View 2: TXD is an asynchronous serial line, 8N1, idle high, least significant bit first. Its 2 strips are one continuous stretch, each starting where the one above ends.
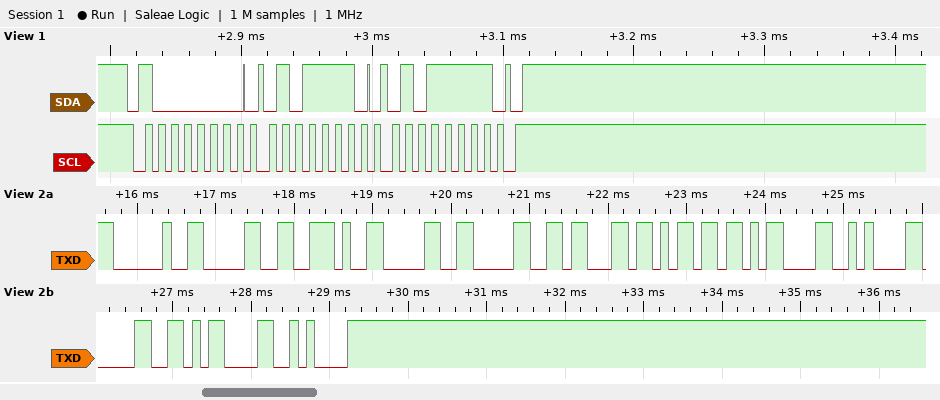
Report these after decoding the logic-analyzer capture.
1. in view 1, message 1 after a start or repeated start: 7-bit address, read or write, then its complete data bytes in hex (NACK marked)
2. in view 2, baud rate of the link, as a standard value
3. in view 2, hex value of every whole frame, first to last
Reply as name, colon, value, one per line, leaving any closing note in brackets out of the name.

in view 1, message 1 after a start or repeated start: 7-bit address, read or write, then its complete data bytes in hex: 0x40 write: 5E 5F
in view 2, baud rate of the link, as a standard value: 9600 baud
in view 2, hex value of every whole frame, first to last: 0x20 0x30 0x2E 0x30 0x30 0x63 0x6D 0x0D 0x0A 0x30 0x0D 0x0A
